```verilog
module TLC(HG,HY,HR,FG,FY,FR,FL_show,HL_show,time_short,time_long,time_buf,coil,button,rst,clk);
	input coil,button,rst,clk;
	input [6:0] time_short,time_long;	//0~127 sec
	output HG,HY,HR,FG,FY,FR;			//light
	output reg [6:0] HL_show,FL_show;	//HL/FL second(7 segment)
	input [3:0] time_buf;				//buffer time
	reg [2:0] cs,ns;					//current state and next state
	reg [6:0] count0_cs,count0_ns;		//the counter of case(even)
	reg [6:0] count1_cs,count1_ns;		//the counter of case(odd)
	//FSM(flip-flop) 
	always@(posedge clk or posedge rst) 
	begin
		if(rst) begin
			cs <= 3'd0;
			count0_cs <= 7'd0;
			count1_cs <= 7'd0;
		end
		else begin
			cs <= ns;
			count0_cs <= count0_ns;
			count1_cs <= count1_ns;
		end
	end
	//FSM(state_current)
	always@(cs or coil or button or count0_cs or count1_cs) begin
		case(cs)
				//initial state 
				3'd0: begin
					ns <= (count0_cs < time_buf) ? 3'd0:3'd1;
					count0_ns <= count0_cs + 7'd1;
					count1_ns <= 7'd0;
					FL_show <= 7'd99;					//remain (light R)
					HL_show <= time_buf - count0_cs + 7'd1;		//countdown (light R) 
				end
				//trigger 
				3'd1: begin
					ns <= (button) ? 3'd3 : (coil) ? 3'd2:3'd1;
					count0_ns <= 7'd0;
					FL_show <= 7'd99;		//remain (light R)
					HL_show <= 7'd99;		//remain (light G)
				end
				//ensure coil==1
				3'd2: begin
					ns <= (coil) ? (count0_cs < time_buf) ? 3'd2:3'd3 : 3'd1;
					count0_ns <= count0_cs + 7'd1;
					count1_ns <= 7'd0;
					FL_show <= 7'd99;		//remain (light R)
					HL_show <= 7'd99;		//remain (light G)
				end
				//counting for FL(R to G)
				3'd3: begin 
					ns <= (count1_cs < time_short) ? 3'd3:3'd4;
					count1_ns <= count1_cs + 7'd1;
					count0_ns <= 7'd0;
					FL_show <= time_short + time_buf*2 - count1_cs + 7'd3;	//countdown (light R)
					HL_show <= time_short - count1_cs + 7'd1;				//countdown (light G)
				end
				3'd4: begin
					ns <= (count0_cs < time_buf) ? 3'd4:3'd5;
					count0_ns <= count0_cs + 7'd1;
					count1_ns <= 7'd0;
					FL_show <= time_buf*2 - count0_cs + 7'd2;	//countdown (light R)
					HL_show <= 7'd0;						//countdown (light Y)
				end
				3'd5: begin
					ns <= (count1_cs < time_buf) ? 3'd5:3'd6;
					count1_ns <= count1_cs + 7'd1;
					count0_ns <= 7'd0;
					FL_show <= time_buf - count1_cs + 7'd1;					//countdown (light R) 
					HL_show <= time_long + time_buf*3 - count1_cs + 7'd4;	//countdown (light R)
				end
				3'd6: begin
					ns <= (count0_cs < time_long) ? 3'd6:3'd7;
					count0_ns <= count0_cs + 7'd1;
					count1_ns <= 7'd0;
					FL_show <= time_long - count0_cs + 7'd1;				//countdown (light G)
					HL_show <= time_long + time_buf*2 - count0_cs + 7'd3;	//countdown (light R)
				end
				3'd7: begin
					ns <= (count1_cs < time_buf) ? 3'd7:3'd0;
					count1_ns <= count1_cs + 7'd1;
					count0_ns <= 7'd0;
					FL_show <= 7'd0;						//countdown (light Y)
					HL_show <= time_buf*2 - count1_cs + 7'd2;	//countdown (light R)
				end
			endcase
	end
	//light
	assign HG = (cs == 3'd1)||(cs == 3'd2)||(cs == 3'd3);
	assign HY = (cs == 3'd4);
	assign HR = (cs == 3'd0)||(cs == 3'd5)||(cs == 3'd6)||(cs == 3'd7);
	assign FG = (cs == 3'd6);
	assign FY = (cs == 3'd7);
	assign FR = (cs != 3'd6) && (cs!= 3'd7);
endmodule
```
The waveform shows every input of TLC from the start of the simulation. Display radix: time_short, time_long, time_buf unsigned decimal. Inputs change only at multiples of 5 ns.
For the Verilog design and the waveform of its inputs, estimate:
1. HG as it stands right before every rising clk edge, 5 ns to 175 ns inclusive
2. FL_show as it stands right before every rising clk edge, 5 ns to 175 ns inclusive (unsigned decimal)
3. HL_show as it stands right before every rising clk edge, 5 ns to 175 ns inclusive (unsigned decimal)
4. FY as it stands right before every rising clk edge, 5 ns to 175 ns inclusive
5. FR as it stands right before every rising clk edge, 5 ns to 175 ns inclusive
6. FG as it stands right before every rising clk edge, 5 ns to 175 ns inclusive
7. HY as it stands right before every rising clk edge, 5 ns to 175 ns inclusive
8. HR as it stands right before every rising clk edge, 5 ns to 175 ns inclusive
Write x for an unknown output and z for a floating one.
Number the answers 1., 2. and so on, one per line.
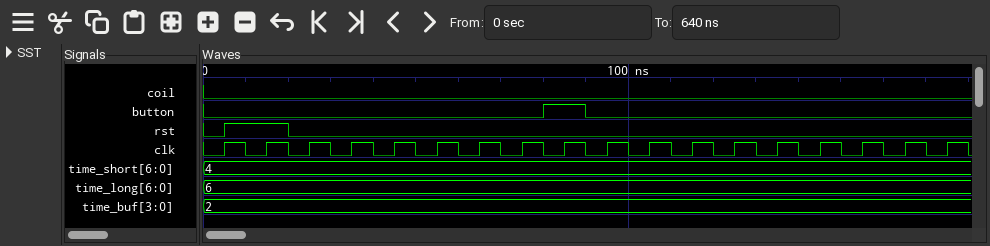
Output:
1. x 0 0 0 0 1 1 1 1 1 1 1 1 1 0 0 0 0
2. x, 99, 99, 99, 99, 99, 99, 99, 99, 11, 10, 9, 8, 7, 6, 5, 4, 3
3. x, 3, 3, 2, 1, 99, 99, 99, 99, 5, 4, 3, 2, 1, 0, 0, 0, 16
4. x 0 0 0 0 0 0 0 0 0 0 0 0 0 0 0 0 0
5. x 1 1 1 1 1 1 1 1 1 1 1 1 1 1 1 1 1
6. x 0 0 0 0 0 0 0 0 0 0 0 0 0 0 0 0 0
7. x 0 0 0 0 0 0 0 0 0 0 0 0 0 1 1 1 0
8. x 1 1 1 1 0 0 0 0 0 0 0 0 0 0 0 0 1
